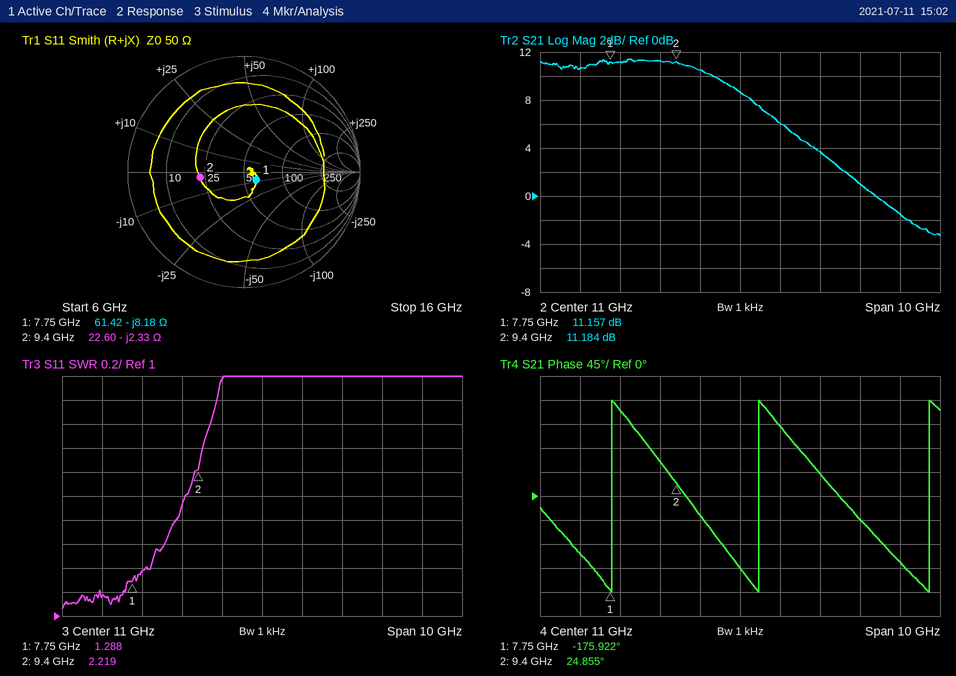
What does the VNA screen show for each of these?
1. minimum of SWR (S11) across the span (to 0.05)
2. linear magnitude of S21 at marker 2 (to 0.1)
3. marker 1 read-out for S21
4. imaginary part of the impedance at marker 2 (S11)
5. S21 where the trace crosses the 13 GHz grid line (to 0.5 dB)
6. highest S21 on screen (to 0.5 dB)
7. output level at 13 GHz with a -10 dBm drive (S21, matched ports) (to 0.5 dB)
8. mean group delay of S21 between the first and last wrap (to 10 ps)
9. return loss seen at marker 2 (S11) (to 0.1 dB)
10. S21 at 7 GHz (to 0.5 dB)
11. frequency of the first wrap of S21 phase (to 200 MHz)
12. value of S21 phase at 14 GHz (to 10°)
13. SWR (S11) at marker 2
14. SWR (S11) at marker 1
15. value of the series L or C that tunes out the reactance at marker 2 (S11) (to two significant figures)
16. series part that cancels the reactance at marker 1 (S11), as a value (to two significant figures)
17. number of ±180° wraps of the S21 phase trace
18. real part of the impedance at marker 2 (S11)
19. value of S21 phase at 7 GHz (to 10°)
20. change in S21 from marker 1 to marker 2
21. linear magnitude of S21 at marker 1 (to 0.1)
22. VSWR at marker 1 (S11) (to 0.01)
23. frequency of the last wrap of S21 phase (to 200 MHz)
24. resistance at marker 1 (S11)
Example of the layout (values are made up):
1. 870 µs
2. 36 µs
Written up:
1. 1.05
2. 3.6
3. 11.157 dB
4. -2.33 Ω
5. 3.5 dB
6. 11.5 dB
7. -6.5 dBm
8. 250 ps
9. 8.4 dB
10. 10.5 dB
11. 7.8 GHz
12. -40°
13. 2.219
14. 1.288
15. 39 pH
16. 170 pH
17. 3
18. 22.60 Ω
19. -110°
20. 0.027 dB
21. 3.6
22. 1.29
23. 15.8 GHz
24. 61.42 Ω
